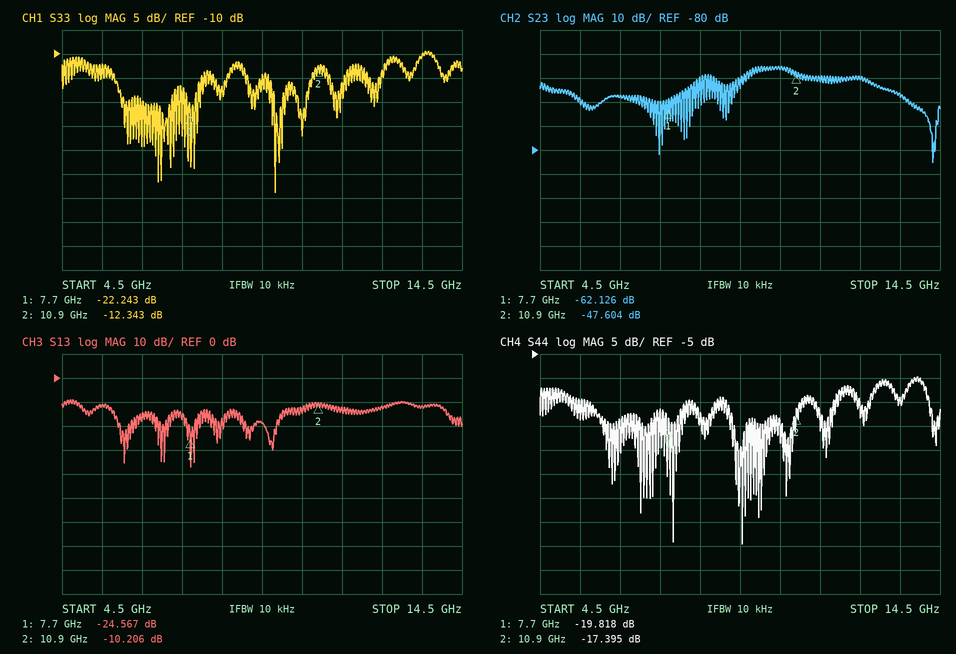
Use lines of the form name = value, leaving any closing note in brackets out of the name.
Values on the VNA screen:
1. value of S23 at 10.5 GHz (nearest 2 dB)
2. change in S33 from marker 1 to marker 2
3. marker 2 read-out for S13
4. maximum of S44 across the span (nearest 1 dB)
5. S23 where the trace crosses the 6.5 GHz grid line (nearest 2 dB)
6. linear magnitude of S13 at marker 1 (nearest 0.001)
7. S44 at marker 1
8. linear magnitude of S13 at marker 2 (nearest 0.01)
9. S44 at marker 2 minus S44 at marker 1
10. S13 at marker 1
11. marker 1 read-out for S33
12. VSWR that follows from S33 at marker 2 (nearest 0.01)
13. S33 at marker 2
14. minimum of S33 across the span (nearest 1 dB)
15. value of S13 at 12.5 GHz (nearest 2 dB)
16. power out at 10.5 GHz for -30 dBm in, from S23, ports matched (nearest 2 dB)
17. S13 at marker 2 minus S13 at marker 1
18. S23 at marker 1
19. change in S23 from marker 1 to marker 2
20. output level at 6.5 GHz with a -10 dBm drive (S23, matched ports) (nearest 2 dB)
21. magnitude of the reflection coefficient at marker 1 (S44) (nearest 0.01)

value of S23 at 10.5 GHz = -46 dB
change in S33 from marker 1 to marker 2 = 9.900 dB
marker 2 read-out for S13 = -10.206 dB
maximum of S44 across the span = -10 dB
S23 where the trace crosses the 6.5 GHz grid line = -58 dB
linear magnitude of S13 at marker 1 = 0.059
S44 at marker 1 = -19.818 dB
linear magnitude of S13 at marker 2 = 0.31
S44 at marker 2 minus S44 at marker 1 = 2.423 dB
S13 at marker 1 = -24.567 dB
marker 1 read-out for S33 = -22.243 dB
VSWR that follows from S33 at marker 2 = 1.64
S33 at marker 2 = -12.343 dB
minimum of S33 across the span = -39 dB
value of S13 at 12.5 GHz = -12 dB
power out at 10.5 GHz for -30 dBm in, from S23, ports matched = -76 dBm
S13 at marker 2 minus S13 at marker 1 = 14.361 dB
S23 at marker 1 = -62.126 dB
change in S23 from marker 1 to marker 2 = 14.522 dB
output level at 6.5 GHz with a -10 dBm drive (S23, matched ports) = -68 dBm
magnitude of the reflection coefficient at marker 1 (S44) = 0.10
